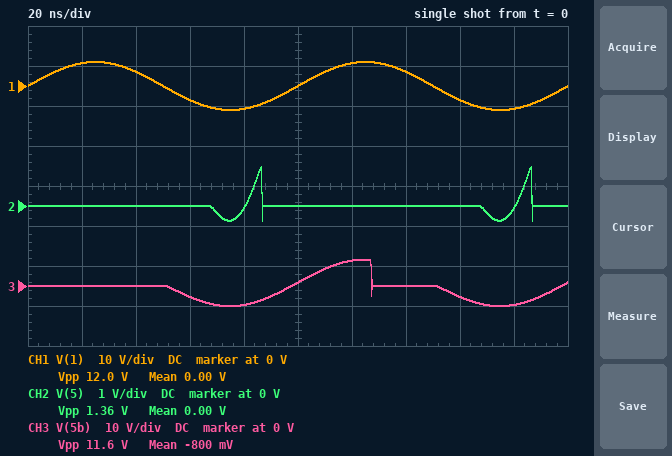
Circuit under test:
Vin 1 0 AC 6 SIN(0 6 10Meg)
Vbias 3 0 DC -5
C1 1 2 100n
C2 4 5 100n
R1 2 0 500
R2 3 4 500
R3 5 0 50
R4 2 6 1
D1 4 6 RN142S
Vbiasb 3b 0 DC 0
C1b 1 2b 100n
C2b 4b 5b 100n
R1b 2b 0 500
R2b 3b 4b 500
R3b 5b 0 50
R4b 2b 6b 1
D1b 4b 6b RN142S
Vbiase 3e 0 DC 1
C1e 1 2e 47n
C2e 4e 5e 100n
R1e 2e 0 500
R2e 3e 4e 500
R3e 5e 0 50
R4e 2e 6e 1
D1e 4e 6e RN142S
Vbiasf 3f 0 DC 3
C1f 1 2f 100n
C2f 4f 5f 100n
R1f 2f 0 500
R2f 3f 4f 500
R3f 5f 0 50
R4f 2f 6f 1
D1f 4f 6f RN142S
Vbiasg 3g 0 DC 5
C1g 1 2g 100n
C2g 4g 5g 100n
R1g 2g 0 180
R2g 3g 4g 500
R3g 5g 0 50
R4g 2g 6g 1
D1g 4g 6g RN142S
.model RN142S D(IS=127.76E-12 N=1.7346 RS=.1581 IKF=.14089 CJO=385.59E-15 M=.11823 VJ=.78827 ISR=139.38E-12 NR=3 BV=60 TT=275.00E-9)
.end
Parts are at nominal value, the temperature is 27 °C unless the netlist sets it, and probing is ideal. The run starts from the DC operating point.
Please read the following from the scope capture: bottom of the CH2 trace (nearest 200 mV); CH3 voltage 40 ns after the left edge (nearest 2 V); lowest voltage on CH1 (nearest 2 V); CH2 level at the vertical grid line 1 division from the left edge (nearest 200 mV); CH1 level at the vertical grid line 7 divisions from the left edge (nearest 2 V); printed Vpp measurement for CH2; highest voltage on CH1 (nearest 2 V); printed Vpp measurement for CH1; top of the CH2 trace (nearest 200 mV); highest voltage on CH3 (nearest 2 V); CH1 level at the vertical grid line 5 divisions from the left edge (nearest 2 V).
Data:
-400 mV
0 V
-6 V
0 V
4 V
1.36 V
6 V
12.0 V
1.0 V
6 V
0 V
